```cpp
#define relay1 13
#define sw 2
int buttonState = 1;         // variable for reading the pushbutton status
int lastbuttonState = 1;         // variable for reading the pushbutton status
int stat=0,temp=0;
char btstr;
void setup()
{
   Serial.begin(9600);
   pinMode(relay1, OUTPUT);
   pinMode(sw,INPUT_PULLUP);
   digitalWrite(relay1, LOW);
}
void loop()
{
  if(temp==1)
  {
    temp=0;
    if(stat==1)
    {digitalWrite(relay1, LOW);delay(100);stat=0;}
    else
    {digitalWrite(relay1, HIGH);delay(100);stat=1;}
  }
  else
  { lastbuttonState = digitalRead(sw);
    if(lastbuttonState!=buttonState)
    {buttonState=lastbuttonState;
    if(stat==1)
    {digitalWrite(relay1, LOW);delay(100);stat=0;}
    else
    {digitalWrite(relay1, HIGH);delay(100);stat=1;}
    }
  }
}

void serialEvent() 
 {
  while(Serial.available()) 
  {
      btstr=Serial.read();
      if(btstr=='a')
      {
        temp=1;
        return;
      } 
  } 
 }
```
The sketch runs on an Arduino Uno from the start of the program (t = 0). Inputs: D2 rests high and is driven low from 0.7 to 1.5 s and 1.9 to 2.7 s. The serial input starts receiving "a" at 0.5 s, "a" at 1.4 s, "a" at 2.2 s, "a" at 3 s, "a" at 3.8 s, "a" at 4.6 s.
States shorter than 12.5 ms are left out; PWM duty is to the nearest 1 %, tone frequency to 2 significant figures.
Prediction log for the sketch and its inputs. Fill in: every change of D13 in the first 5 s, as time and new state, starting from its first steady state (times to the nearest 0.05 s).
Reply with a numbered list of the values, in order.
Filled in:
1. 0 s low; 0.5 s high; 0.7 s low; 1.4 s high; 1.5 s low; 1.9 s high; 2.2 s low; 2.7 s high; 3 s low; 3.8 s high; 4.6 s low
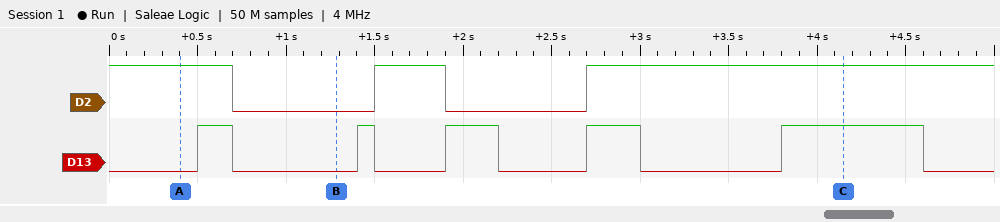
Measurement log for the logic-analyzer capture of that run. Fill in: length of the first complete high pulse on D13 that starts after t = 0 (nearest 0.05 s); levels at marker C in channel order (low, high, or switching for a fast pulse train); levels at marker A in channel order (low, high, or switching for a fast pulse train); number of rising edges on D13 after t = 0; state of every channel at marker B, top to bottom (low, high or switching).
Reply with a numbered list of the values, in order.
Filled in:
1. 0.20 s
2. D2 high, D13 high
3. D2 high, D13 low
4. 5
5. D2 low, D13 low
